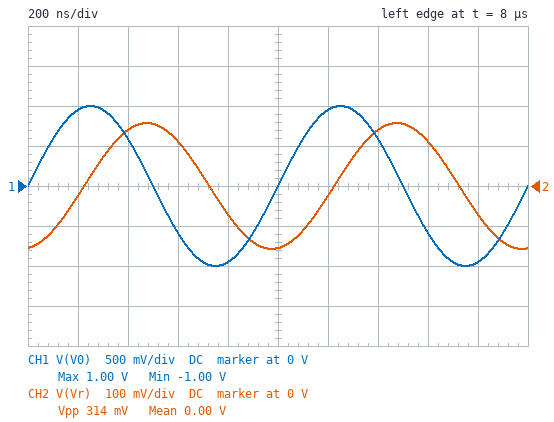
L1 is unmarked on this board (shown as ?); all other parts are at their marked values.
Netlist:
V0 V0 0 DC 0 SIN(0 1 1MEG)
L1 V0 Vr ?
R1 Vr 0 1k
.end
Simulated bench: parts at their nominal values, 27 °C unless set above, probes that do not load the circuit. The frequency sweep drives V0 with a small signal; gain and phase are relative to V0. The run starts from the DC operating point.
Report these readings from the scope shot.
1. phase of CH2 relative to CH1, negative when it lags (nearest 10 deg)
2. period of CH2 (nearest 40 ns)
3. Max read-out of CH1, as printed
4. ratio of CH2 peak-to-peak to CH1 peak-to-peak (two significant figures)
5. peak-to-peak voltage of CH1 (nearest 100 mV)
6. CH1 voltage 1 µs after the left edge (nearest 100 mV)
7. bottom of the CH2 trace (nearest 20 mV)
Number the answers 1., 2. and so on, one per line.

1. -80 deg
2. 1.00 µs
3. 1.00 V
4. 0.16
5. 2.0 V
6. 0 V
7. -160 mV
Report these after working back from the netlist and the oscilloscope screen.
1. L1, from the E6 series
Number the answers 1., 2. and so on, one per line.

1. 1 mH
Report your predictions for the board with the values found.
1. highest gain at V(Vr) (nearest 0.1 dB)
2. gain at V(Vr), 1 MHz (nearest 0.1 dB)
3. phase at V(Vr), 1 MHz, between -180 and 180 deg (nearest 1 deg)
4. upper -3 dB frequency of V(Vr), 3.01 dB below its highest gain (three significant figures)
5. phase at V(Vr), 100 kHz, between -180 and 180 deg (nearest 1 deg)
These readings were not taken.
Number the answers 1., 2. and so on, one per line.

1. 0 dB
2. -16.1 dB
3. -81 deg
4. 159 kHz
5. -32 deg
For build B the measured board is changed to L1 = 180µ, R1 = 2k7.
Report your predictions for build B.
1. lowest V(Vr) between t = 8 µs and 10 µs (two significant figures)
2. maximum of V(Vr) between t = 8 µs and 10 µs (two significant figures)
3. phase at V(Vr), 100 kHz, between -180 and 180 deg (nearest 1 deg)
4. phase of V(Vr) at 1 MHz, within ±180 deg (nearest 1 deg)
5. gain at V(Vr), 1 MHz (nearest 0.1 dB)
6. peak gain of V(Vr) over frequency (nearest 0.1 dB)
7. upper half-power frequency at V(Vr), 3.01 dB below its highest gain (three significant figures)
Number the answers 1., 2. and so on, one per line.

1. -920 mV
2. 920 mV
3. -2 deg
4. -23 deg
5. -0.7 dB
6. 0 dB
7. 2.39 MHz
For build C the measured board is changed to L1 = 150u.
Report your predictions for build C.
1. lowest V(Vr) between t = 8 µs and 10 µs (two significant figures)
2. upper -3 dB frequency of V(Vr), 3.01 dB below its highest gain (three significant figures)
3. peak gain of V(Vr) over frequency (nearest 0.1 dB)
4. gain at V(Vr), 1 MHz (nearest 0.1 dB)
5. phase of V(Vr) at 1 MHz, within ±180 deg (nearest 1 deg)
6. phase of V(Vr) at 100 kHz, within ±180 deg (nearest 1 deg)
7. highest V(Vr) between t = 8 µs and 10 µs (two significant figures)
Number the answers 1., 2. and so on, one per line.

1. -730 mV
2. 1.06 MHz
3. 0 dB
4. -2.8 dB
5. -43 deg
6. -5 deg
7. 730 mV
